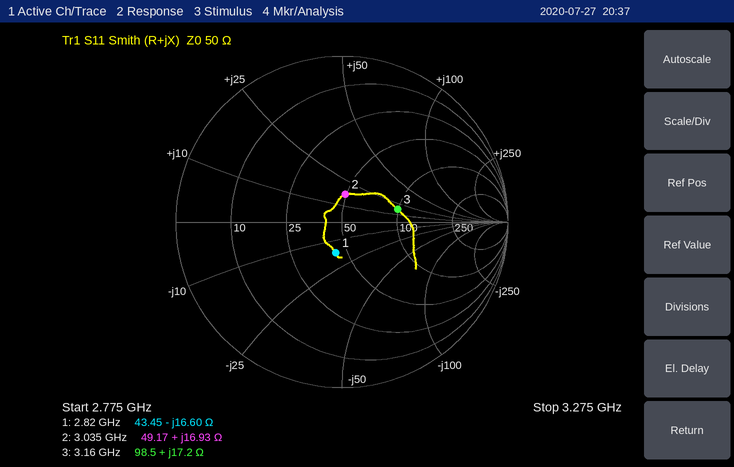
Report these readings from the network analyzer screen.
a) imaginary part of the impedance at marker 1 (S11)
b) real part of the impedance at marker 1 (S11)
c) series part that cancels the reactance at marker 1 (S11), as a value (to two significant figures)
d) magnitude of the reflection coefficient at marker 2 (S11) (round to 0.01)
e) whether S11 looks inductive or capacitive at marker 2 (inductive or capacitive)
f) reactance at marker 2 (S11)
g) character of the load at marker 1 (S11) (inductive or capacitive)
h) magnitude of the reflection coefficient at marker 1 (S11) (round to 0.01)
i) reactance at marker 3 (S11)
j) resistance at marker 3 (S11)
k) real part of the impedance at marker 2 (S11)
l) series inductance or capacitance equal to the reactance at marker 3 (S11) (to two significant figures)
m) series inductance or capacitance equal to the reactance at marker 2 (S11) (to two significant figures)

-16.60 Ω
43.45 Ω
940 pH
0.17
inductive
+16.93 Ω
capacitive
0.19
+17.2 Ω
98.5 Ω
49.17 Ω
870 pH
890 pH
